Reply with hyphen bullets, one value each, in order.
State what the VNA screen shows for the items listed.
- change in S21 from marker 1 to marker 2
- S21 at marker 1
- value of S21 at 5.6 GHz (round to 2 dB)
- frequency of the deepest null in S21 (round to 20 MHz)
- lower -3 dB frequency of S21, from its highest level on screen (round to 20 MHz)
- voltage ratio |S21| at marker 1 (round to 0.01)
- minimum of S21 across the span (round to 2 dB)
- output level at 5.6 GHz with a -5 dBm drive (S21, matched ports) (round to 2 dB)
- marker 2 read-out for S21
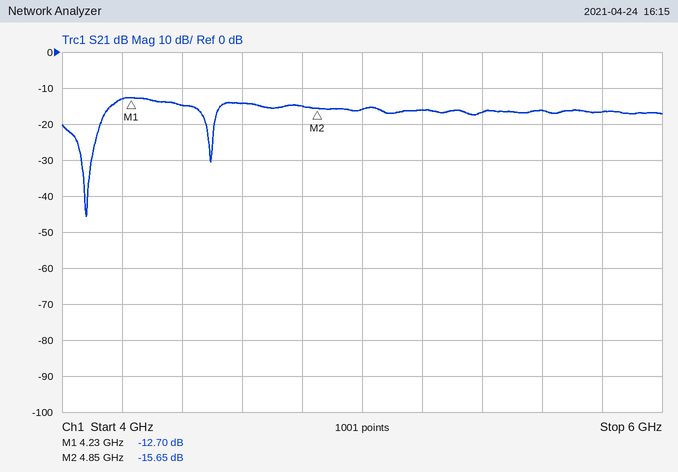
- -2.95 dB
- -12.70 dB
- -16 dB
- 4.08 GHz
- 4.16 GHz
- 0.23
- -46 dB
- -22 dBm
- -15.65 dB
